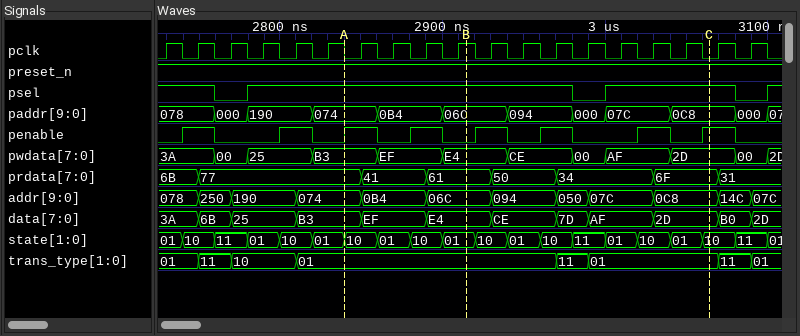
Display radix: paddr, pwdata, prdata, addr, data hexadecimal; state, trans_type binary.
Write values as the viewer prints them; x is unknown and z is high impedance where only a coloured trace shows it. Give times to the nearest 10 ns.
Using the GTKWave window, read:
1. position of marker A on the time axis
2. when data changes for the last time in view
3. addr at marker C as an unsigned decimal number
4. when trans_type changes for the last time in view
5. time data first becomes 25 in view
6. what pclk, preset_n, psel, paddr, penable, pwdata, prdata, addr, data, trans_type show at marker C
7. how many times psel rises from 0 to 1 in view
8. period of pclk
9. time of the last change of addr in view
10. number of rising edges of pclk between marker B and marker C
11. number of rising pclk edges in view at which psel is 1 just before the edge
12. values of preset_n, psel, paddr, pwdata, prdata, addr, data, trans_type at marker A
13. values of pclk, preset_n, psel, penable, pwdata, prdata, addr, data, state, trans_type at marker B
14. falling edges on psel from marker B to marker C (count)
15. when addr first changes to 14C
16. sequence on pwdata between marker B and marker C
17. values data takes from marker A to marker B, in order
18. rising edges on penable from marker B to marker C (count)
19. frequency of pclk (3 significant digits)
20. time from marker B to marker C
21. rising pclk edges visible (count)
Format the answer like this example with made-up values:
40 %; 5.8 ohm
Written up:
2840 ns; 3090 ns; 200; 3090 ns; 2770 ns; pclk=0, preset_n=1, psel=1, paddr=0C8, penable=1, pwdata=2D, prdata=6F, addr=0C8, data=2D, trans_type=01; 3; 20 ns; 3090 ns; 7; 16; preset_n=1, psel=1, paddr=074, pwdata=B3, prdata=77, addr=074, data=B3, trans_type=01; pclk=1, preset_n=1, psel=1, penable=0, pwdata=E4, prdata=61, addr=06C, data=E4, state=01, trans_type=01; 1; 3070 ns; E4, CE, 00, AF, 2D; B3, EF, E4; 4; 50.0 MHz; 150 ns; 19
